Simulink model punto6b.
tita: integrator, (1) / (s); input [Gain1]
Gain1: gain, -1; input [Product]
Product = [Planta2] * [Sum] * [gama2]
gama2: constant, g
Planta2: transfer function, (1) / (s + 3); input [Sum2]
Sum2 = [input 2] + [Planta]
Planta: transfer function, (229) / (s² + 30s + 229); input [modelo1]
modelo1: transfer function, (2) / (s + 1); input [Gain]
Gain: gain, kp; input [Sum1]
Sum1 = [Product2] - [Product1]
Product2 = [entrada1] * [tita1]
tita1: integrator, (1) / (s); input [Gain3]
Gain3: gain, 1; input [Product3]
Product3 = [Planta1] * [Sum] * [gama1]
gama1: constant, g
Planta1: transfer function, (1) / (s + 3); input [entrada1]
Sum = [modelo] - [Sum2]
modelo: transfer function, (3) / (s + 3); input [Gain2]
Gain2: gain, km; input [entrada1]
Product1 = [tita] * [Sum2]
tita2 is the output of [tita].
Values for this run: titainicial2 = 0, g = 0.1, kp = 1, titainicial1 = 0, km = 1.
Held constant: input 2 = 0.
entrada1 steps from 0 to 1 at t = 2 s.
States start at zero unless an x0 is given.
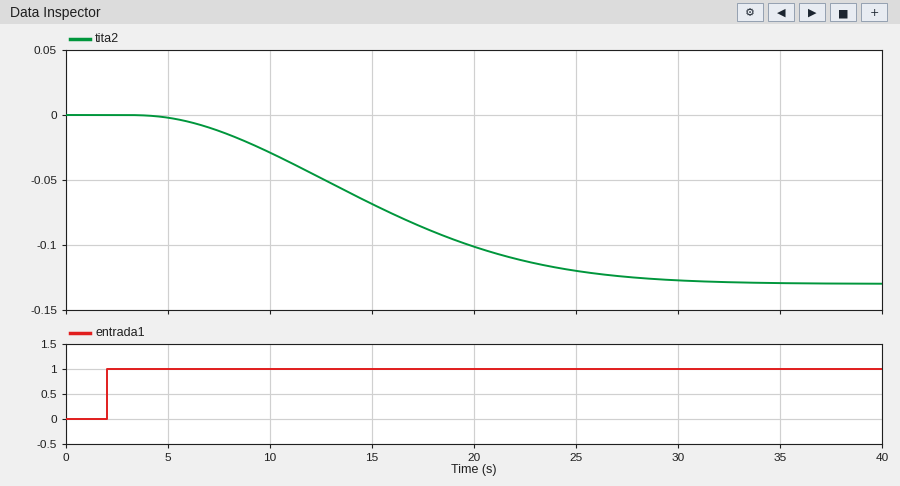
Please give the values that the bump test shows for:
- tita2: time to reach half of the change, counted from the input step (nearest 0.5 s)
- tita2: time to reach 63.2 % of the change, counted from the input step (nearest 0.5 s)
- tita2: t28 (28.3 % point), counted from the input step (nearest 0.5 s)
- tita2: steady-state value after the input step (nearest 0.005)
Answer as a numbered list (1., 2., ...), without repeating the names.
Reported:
1. 12.5 s
2. 15.0 s
3. 9.0 s
4. -0.130
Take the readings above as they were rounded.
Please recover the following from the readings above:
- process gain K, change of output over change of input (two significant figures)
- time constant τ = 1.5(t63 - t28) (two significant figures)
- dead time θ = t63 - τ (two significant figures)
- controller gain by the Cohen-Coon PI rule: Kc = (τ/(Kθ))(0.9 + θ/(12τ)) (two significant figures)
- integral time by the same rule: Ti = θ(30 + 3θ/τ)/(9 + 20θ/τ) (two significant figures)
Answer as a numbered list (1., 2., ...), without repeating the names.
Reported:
1. -0.13
2. 9.0 s
3. 6.0 s
4. -11
5. 8.6 s
